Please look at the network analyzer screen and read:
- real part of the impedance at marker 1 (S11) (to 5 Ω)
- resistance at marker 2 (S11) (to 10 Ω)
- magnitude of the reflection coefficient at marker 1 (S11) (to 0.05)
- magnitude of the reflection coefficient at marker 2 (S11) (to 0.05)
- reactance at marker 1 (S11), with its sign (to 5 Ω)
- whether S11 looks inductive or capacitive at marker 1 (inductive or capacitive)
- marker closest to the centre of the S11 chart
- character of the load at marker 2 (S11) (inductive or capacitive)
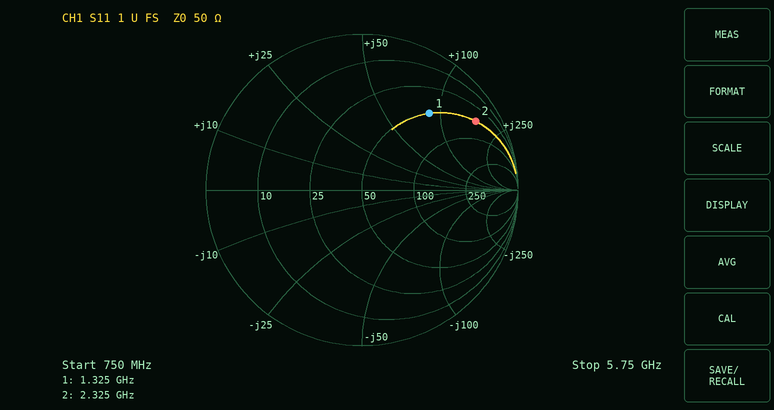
50 Ω
50 Ω
0.65
0.85
+85 Ω
inductive
marker 1
inductive
